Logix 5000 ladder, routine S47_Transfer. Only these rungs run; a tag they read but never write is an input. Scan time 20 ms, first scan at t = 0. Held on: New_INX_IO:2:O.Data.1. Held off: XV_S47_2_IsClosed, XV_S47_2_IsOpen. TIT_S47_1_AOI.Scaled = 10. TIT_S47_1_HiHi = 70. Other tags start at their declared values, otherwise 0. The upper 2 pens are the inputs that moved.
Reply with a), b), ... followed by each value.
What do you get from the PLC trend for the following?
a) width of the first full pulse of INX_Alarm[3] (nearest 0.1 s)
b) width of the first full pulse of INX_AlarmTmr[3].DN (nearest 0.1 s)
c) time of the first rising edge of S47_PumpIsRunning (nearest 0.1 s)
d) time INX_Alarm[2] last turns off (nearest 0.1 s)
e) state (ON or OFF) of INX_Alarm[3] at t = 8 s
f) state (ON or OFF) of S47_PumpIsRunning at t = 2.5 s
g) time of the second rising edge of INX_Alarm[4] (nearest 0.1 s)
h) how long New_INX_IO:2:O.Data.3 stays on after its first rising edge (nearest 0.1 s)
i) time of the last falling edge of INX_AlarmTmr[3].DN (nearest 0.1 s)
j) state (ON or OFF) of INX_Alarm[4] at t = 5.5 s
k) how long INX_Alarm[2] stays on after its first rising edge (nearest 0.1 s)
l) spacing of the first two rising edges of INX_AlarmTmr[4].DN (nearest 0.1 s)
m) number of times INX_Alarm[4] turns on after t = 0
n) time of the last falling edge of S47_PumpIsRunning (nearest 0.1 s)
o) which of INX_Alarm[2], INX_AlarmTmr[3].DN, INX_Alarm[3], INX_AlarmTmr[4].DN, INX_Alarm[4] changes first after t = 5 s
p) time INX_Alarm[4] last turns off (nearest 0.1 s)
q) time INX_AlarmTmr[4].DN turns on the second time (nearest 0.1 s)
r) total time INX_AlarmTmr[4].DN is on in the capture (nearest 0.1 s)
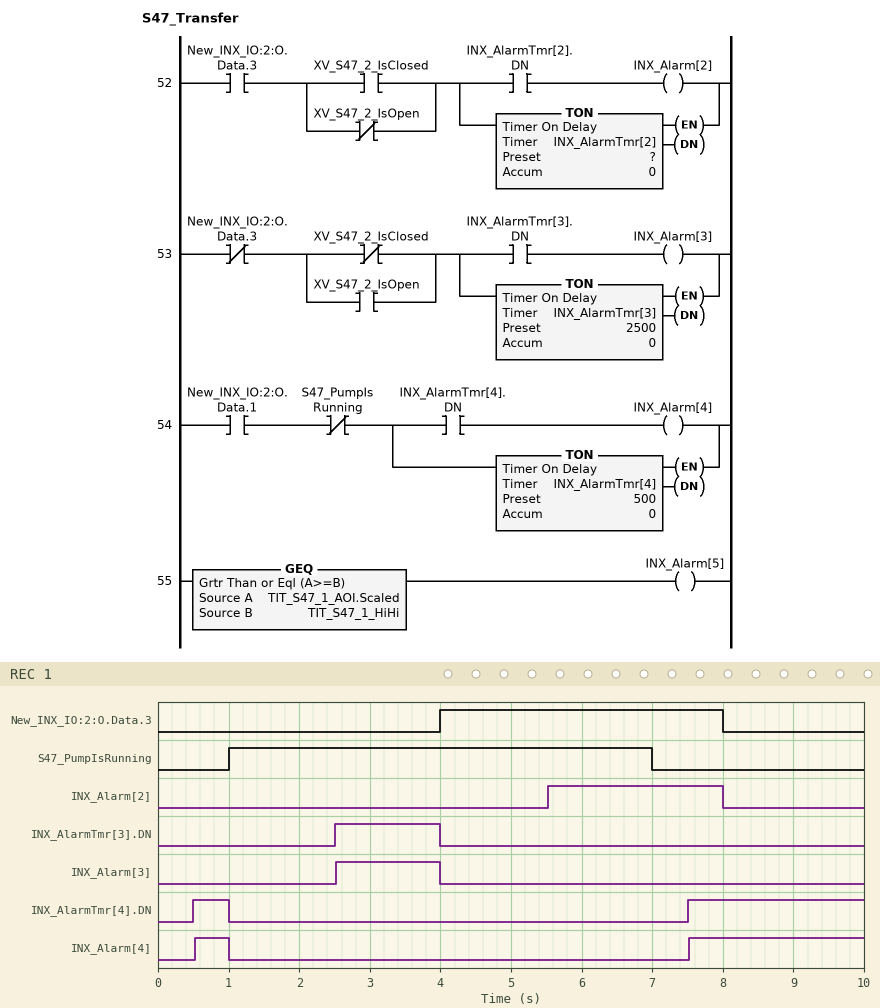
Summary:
a) 1.5 s
b) 1.5 s
c) 1.0 s
d) 8.0 s
e) OFF
f) ON
g) 7.5 s
h) 4.0 s
i) 4.0 s
j) OFF
k) 2.5 s
l) 7.0 s
m) 2
n) 7.0 s
o) INX_Alarm[2]
p) 1.0 s
q) 7.5 s
r) 3.0 s
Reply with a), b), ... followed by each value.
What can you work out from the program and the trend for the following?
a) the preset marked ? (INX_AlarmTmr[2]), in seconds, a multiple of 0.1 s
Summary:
a) 1.5 s
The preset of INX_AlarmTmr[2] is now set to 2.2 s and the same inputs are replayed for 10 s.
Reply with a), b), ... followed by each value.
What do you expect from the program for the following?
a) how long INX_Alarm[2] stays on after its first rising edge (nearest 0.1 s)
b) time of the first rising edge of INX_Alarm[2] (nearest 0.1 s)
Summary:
a) 1.8 s
b) 6.2 s
